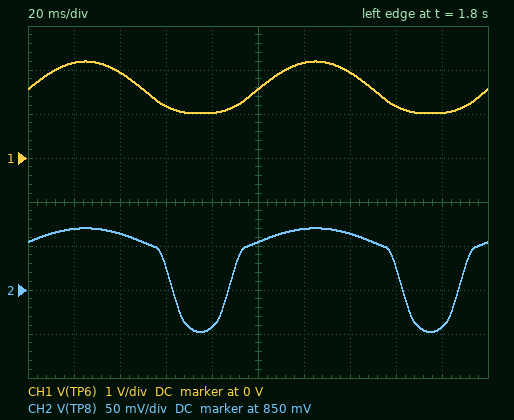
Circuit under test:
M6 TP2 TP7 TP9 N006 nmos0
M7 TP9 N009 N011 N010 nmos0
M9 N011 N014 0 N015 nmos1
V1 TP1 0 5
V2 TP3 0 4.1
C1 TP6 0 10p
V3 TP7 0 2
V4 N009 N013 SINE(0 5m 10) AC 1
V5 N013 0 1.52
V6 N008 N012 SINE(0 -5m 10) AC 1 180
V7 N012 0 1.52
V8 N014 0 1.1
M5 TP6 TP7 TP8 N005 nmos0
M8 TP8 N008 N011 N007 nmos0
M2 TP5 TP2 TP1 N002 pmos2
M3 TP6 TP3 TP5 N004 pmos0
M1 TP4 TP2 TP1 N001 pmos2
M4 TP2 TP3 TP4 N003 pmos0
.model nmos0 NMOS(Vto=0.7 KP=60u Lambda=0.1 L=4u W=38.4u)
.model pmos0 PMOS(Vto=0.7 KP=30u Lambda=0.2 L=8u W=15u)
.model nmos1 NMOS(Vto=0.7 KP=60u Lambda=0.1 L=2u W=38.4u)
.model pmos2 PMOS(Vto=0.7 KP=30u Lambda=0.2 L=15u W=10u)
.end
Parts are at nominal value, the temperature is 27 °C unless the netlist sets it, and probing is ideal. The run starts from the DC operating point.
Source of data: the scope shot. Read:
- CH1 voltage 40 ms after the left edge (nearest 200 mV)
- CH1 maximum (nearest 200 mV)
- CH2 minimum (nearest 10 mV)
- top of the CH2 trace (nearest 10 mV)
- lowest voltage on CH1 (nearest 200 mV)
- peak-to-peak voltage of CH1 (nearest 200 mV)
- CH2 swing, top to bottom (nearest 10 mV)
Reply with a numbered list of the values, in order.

1. 2.0 V
2. 2.2 V
3. 800 mV
4. 920 mV
5. 1.0 V
6. 1.2 V
7. 120 mV
